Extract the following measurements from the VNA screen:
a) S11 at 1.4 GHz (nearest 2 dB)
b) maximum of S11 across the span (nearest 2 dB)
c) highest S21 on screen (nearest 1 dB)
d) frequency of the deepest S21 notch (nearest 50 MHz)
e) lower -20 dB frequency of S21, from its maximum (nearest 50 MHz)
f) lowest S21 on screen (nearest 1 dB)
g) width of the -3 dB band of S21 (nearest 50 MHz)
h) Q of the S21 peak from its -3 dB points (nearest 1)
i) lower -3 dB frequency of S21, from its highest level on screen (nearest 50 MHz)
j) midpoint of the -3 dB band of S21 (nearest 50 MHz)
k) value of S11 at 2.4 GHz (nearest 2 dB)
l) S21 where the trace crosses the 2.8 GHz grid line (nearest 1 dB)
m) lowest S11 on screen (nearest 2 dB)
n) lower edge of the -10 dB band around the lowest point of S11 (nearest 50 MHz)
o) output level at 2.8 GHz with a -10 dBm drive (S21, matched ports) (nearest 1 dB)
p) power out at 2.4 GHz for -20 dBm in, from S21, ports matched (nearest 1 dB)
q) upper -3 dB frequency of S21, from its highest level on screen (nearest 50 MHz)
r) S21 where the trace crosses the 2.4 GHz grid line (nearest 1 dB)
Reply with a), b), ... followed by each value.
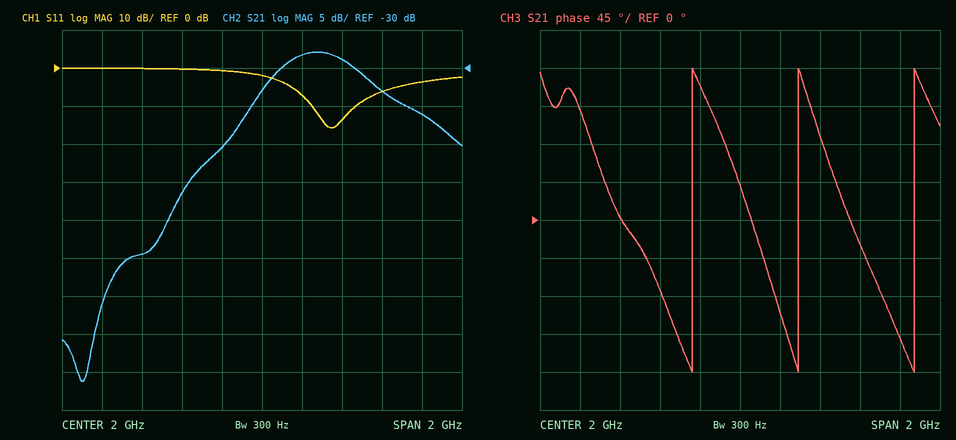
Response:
a) 0 dB
b) 0 dB
c) -28 dB
d) 1.10 GHz
e) 1.55 GHz
f) -71 dB
g) 450 MHz
h) 5
i) 2.05 GHz
j) 2.30 GHz
k) -14 dB
l) -36 dB
m) -16 dB
n) 2.25 GHz
o) -46 dBm
p) -49 dBm
q) 2.50 GHz
r) -29 dB
